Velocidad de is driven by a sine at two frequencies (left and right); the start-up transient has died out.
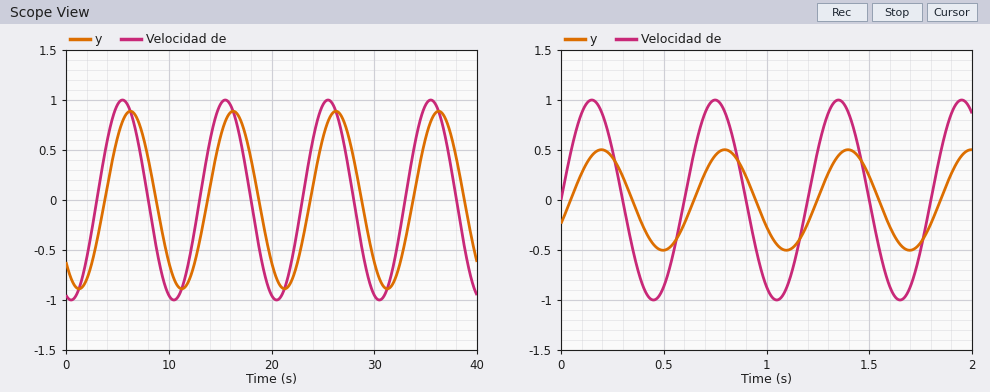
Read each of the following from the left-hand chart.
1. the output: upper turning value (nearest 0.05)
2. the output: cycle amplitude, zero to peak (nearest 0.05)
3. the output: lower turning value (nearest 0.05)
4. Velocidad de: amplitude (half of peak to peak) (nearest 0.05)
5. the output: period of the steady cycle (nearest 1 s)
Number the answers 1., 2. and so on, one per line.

1. 0.90
2. 0.90
3. -0.90
4. 1.00
5. 10 s
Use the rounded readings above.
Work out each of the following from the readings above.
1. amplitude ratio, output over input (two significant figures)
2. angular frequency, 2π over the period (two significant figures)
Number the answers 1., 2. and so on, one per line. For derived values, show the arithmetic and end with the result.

1. 0.9 / 1 = 0.90
2. 2π / 10 = 0.63 rad/s
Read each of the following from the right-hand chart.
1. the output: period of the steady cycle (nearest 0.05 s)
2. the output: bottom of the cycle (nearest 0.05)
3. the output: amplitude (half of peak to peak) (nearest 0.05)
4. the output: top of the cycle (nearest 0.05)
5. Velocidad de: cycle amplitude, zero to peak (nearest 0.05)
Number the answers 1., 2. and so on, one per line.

1. 0.60 s
2. -0.50
3. 0.50
4. 0.50
5. 1.00
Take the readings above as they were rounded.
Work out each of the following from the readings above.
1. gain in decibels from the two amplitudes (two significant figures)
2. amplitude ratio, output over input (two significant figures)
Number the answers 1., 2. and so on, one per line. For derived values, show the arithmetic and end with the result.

1. 20 log10(0.5 / 1) = -6.0 dB
2. 0.5 / 1 = 0.50
